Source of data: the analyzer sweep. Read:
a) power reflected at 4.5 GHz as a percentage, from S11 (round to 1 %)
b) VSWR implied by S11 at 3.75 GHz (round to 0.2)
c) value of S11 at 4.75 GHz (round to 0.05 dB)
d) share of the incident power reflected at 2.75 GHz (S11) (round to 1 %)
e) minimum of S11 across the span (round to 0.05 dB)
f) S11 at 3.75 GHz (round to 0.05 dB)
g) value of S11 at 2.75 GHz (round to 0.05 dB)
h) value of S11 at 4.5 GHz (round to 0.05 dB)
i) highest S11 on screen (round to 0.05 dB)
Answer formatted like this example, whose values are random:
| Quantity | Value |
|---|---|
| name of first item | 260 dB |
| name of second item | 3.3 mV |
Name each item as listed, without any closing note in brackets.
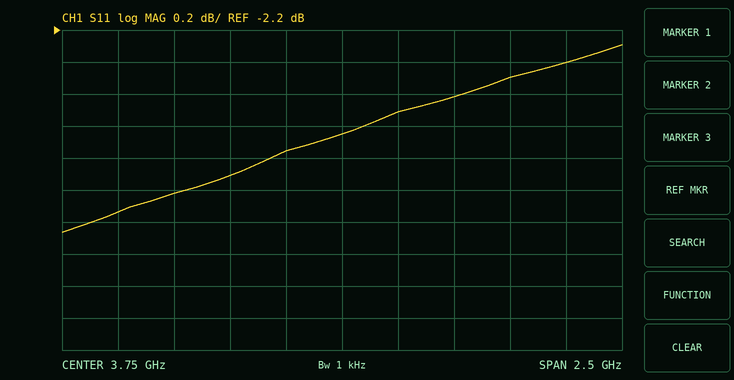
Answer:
| Quantity | Value |
|---|---|
| power reflected at 4.5 GHz as a percentage, from S11 | 56 % |
| VSWR implied by S11 at 3.75 GHz | 6.2 |
| value of S11 at 4.75 GHz | -2.40 dB |
| share of the incident power reflected at 2.75 GHz (S11) | 46 % |
| minimum of S11 across the span | -3.45 dB |
| S11 at 3.75 GHz | -2.85 dB |
| value of S11 at 2.75 GHz | -3.35 dB |
| value of S11 at 4.5 GHz | -2.50 dB |
| highest S11 on screen | -2.30 dB |
